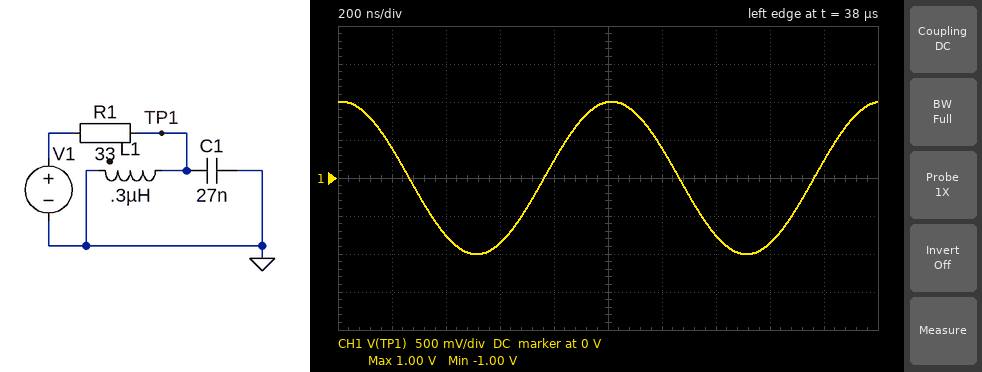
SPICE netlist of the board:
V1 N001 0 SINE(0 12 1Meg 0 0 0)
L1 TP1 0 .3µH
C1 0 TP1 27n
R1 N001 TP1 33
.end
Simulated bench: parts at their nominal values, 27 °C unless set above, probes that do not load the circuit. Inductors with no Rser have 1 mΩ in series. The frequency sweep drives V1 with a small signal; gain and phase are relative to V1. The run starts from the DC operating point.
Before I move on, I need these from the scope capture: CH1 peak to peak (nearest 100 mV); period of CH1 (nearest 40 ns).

2.0 V
1.00 µs
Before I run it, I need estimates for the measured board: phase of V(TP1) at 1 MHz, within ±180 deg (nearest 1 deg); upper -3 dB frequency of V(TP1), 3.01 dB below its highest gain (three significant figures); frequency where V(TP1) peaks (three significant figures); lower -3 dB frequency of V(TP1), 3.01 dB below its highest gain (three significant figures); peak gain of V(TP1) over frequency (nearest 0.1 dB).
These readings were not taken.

85 deg
1.86 MHz
1.77 MHz
1.68 MHz
0 dB
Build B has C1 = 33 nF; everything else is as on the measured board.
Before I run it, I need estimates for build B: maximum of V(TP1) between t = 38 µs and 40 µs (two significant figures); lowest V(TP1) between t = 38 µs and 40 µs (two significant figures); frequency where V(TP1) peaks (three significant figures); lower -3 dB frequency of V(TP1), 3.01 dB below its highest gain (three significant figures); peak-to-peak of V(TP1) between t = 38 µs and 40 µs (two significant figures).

1.1 V
-1.1 V
1.60 MHz
1.53 MHz
2.2 V
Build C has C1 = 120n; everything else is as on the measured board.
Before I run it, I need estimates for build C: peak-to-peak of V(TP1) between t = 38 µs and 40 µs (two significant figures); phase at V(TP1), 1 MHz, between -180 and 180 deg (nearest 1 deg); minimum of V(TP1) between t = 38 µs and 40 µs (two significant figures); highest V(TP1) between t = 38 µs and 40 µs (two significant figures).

3.2 V
-82 deg
-1.6 V
1.6 V
